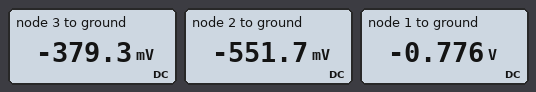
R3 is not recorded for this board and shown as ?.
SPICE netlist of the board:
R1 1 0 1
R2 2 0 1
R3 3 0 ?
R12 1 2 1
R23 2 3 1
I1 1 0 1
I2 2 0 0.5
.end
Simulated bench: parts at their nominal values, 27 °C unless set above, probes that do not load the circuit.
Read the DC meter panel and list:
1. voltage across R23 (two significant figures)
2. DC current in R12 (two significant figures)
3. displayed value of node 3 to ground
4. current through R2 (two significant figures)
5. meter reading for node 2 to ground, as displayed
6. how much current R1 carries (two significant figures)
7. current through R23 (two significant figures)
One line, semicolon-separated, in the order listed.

170 mV; 220 mA; -379.3 mV; 550 mA; -551.7 mV; 780 mA; 170 mA
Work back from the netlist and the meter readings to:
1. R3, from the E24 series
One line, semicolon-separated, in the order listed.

2.2 Ω
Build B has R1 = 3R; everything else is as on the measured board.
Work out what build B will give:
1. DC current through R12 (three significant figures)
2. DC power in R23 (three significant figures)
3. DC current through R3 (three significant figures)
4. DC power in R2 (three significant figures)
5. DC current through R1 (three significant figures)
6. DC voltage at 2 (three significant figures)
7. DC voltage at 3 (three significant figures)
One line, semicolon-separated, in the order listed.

550 mA; 62.5 mW; 250 mA; 640 mW; 450 mA; -800 mV; -550 mV
